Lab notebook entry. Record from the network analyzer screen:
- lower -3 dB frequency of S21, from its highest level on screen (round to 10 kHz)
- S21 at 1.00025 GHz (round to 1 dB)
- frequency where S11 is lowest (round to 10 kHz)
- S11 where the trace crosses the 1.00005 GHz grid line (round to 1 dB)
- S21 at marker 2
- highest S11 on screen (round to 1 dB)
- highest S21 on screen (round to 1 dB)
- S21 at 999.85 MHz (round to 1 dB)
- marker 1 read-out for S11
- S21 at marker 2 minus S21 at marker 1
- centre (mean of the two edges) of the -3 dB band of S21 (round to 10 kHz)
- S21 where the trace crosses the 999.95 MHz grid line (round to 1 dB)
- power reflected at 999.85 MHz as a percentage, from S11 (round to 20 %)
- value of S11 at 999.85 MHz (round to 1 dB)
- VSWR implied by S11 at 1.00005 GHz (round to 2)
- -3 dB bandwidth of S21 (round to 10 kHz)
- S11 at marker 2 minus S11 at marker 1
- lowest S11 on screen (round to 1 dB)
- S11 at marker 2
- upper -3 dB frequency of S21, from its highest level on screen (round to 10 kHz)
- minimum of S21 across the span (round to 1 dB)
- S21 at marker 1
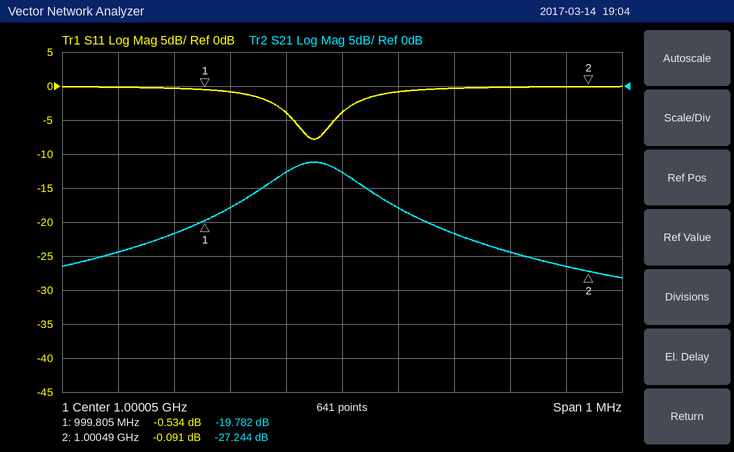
999.92 MHz
-22 dB
1.00000 GHz
-4 dB
-27.244 dB
0 dB
-11 dB
-18 dB
-0.534 dB
-7.462 dB
1.00000 GHz
-13 dB
80 %
-1 dB
4
160 kHz
0.443 dB
-8 dB
-0.091 dB
1.00008 GHz
-28 dB
-19.782 dB
